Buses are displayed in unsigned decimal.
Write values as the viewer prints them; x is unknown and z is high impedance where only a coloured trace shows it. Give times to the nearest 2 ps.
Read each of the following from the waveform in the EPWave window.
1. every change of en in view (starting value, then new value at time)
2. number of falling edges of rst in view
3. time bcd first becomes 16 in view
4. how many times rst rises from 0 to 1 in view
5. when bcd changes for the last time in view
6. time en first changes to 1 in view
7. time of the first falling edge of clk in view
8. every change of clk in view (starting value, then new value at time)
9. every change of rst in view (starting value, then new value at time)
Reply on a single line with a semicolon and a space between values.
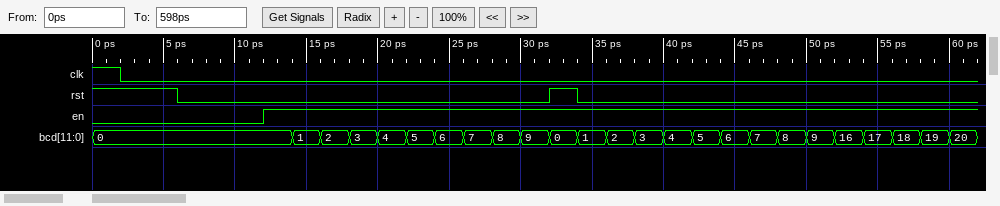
0, 1 at 12 ps; 2; 52 ps; 1; 60 ps; 12 ps; 2 ps; 1, 0 at 2 ps; 1, 0 at 6 ps, 1 at 32 ps, 0 at 34 ps
